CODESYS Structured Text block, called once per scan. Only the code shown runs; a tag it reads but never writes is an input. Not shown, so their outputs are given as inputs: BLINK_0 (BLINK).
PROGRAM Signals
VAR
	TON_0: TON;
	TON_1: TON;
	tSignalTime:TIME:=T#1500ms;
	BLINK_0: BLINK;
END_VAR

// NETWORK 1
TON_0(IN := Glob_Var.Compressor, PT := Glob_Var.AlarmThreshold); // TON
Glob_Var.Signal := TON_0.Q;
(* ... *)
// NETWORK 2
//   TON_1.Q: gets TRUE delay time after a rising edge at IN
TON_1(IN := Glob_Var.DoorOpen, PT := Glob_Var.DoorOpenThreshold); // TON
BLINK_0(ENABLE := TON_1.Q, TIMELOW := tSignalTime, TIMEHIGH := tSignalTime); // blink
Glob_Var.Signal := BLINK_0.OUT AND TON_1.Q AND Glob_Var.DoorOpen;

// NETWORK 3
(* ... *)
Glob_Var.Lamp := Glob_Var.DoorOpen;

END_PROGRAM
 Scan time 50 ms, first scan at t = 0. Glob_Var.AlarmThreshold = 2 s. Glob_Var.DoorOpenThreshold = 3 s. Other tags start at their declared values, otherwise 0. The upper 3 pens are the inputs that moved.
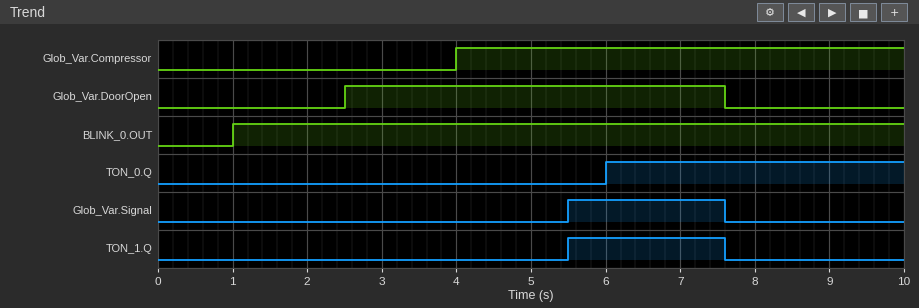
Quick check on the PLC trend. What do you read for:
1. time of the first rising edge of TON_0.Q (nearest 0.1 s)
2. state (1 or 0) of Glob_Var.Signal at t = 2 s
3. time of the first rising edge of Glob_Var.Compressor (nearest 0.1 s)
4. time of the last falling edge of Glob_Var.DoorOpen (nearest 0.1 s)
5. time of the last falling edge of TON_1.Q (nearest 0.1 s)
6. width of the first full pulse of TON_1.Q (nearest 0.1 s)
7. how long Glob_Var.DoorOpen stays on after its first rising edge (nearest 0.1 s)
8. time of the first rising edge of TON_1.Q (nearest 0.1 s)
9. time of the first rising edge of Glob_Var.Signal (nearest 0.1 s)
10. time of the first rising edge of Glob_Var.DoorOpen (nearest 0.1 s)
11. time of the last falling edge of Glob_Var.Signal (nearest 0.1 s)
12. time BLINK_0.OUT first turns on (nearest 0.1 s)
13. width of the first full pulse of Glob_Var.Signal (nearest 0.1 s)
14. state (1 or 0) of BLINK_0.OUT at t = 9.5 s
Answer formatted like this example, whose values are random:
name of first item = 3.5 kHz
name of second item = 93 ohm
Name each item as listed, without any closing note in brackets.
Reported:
time of the first rising edge of TON_0.Q = 6.0 s
state (1 or 0) of Glob_Var.Signal at t = 2 s = 0
time of the first rising edge of Glob_Var.Compressor = 4.0 s
time of the last falling edge of Glob_Var.DoorOpen = 7.6 s
time of the last falling edge of TON_1.Q = 7.6 s
width of the first full pulse of TON_1.Q = 2.1 s
how long Glob_Var.DoorOpen stays on after its first rising edge = 5.1 s
time of the first rising edge of TON_1.Q = 5.5 s
time of the first rising edge of Glob_Var.Signal = 5.5 s
time of the first rising edge of Glob_Var.DoorOpen = 2.5 s
time of the last falling edge of Glob_Var.Signal = 7.6 s
time BLINK_0.OUT first turns on = 1.0 s
width of the first full pulse of Glob_Var.Signal = 2.1 s
state (1 or 0) of BLINK_0.OUT at t = 9.5 s = 1
